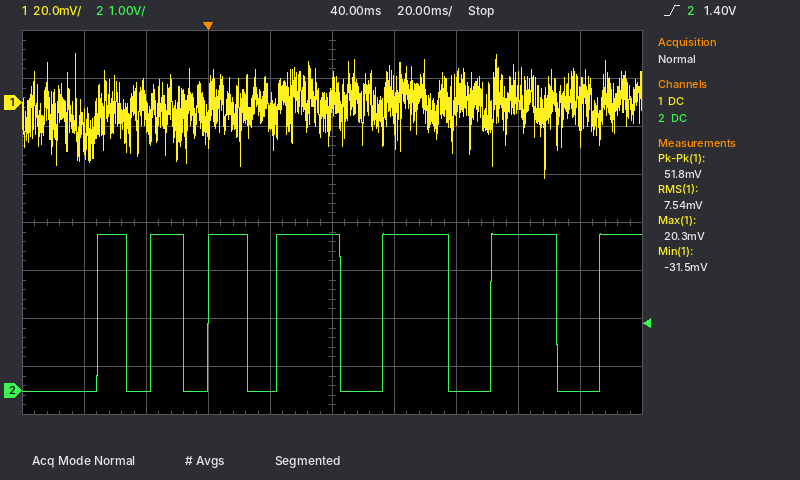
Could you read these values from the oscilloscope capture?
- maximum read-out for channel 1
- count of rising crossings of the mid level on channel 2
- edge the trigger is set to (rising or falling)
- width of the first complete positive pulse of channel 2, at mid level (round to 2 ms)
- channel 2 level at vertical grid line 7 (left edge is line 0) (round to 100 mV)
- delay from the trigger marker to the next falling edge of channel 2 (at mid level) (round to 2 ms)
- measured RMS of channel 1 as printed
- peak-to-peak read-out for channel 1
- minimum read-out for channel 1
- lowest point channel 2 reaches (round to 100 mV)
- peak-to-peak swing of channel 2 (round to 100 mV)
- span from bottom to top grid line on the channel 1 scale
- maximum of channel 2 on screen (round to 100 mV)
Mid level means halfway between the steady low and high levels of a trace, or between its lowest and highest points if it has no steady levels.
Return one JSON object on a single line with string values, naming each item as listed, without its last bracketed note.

{"maximum read-out for channel 1": "20.3 mV", "count of rising crossings of the mid level on channel 2": "7", "edge the trigger is set to": "rising", "width of the first complete positive pulse of channel 2, at mid level": "10 ms", "channel 2 level at vertical grid line 7 (left edge is line 0)": "0.0 V", "delay from the trigger marker to the next falling edge of channel 2 (at mid level)": "12 ms", "measured RMS of channel 1 as printed": "7.54 mV", "peak-to-peak read-out for channel 1": "51.8 mV", "minimum read-out for channel 1": "-31.5 mV", "lowest point channel 2 reaches": "0.0 V", "peak-to-peak swing of channel 2": "3.3 V", "span from bottom to top grid line on the channel 1 scale": "160 mV", "maximum of channel 2 on screen": "3.3 V"}
